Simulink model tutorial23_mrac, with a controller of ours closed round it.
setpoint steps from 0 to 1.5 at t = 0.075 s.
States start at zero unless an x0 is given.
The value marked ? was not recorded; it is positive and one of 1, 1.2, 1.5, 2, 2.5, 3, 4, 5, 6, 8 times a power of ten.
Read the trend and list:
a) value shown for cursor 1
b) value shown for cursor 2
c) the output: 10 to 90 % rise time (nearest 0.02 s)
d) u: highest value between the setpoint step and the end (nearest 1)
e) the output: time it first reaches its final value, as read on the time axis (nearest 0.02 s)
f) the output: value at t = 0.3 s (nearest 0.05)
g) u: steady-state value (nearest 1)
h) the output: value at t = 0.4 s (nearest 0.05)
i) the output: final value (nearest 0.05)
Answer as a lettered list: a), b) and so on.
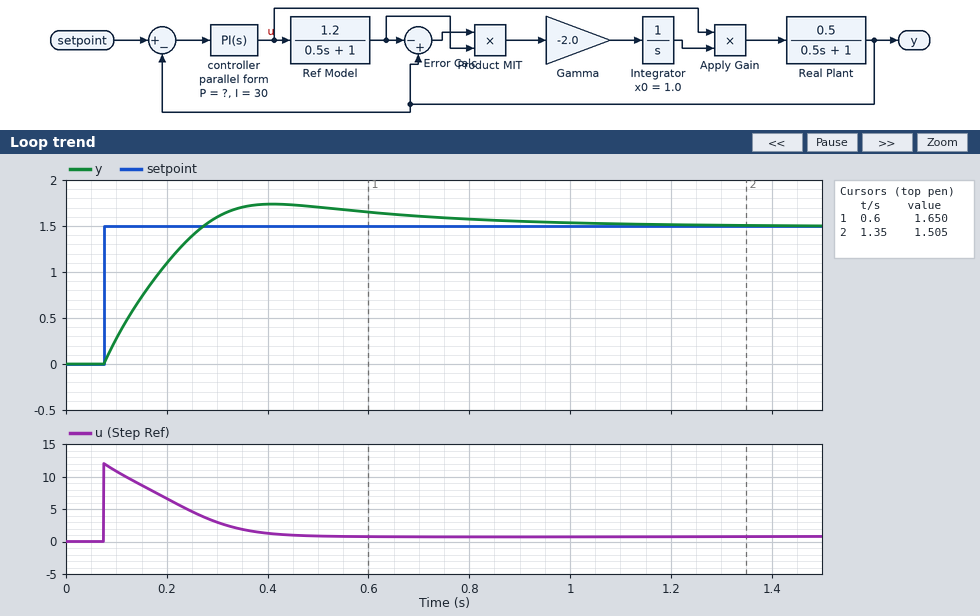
a) 1.650
b) 1.505
c) 0.16 s
d) 12
e) 0.28 s
f) 1.60
g) 1
h) 1.75
i) 1.50
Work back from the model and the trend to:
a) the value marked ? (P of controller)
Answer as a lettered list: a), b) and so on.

a) 8
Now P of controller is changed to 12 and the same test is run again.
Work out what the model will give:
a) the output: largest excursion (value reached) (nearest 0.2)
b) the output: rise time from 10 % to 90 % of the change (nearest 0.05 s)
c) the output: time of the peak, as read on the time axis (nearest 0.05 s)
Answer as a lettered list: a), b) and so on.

a) 1.6
b) 0.15 s
c) 0.40 s
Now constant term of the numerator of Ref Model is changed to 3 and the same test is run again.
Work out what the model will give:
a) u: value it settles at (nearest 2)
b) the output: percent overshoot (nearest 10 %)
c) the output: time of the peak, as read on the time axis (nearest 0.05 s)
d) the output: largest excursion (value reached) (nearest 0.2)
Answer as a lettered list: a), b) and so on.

a) 0
b) 20 %
c) 0.30 s
d) 1.8
